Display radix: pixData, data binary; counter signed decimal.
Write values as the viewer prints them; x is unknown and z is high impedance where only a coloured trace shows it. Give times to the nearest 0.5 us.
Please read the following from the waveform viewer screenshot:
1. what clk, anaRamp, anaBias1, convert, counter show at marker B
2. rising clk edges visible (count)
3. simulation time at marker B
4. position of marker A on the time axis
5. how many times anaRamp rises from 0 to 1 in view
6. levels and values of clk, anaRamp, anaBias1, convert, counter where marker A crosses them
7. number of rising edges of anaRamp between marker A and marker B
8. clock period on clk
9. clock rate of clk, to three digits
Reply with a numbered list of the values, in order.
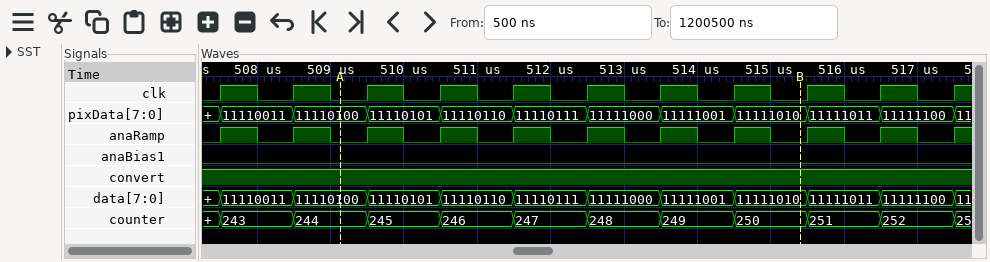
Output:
1. clk=0, anaRamp=0, anaBias1=0, convert=1, counter=250
2. 11
3. 515.5 us
4. 509 us
5. 11
6. clk=0, anaRamp=0, anaBias1=0, convert=1, counter=244
7. 6
8. 1 us
9. 1.00 MHz
